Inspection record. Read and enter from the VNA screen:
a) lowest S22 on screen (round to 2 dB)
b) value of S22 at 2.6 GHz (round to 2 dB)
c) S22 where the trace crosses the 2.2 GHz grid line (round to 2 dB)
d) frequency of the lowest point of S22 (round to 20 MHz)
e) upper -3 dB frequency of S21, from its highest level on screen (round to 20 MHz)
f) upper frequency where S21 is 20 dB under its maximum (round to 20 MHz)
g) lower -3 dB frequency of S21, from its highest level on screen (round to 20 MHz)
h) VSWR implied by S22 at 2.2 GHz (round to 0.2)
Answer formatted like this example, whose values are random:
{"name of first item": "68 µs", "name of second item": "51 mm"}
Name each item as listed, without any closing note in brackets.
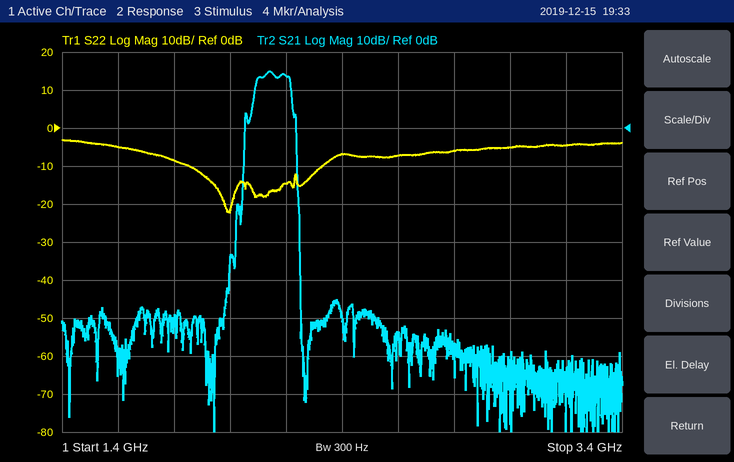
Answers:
{"lowest S22 on screen": "-22 dB", "value of S22 at 2.6 GHz": "-8 dB", "S22 where the trace crosses the 2.2 GHz grid line": "-14 dB", "frequency of the lowest point of S22": "2.00 GHz", "upper -3 dB frequency of S21, from its highest level on screen": "2.22 GHz", "upper frequency where S21 is 20 dB under its maximum": "2.24 GHz", "lower -3 dB frequency of S21, from its highest level on screen": "2.10 GHz", "VSWR implied by S22 at 2.2 GHz": "1.4"}
